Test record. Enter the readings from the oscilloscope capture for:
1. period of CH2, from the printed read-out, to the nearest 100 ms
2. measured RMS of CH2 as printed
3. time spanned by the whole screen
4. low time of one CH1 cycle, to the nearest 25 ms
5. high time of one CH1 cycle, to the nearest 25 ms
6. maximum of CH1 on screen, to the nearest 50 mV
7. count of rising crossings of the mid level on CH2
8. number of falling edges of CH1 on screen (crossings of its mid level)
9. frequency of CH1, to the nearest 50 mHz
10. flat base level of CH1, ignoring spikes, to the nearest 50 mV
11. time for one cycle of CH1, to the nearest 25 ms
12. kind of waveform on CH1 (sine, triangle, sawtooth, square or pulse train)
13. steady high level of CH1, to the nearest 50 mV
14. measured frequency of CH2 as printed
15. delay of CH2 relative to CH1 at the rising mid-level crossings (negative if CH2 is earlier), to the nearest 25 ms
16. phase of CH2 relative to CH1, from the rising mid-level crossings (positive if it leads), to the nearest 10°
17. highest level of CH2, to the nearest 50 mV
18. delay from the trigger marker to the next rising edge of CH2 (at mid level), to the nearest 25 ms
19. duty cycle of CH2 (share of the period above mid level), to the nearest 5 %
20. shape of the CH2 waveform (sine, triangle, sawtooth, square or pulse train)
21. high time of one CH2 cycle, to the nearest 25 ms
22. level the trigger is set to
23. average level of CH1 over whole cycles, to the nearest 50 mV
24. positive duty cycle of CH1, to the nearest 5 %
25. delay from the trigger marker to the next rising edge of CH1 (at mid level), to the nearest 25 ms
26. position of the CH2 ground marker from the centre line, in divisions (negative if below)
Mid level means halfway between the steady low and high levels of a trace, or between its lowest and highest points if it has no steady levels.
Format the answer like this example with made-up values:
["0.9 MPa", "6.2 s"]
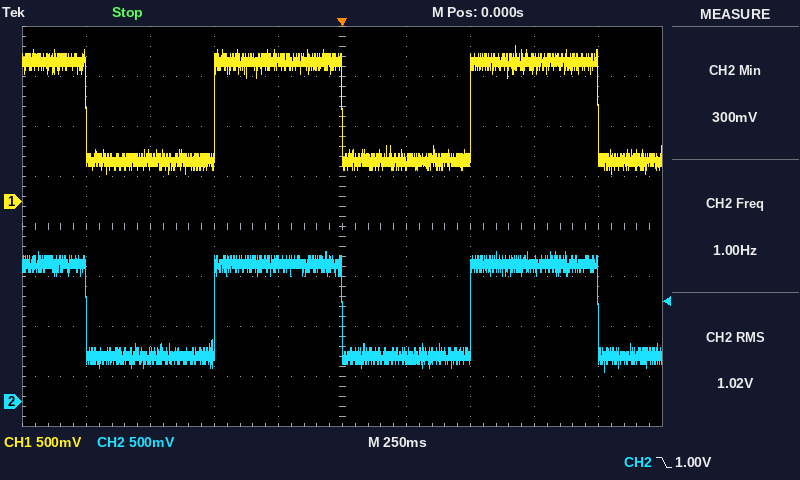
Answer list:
["1.0 s", "1.02 V", "2.5 s", "500 ms", "500 ms", "1.55 V", "2", "3", "1.00 Hz", "400 mV", "1.000 s", "square", "1.40 V", "1.00 Hz", "0 ms", "0°", "1.50 V", "500 ms", "50 %", "square", "500 ms", "1.00 V", "900 mV", "50 %", "500 ms", "-3.5 div"]
